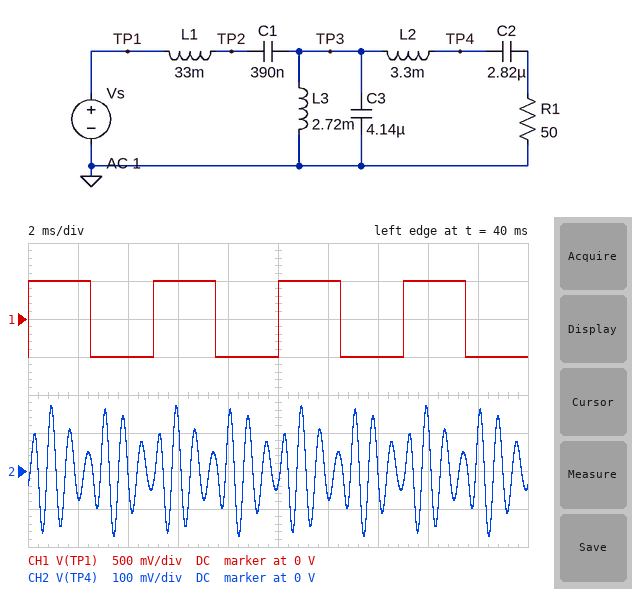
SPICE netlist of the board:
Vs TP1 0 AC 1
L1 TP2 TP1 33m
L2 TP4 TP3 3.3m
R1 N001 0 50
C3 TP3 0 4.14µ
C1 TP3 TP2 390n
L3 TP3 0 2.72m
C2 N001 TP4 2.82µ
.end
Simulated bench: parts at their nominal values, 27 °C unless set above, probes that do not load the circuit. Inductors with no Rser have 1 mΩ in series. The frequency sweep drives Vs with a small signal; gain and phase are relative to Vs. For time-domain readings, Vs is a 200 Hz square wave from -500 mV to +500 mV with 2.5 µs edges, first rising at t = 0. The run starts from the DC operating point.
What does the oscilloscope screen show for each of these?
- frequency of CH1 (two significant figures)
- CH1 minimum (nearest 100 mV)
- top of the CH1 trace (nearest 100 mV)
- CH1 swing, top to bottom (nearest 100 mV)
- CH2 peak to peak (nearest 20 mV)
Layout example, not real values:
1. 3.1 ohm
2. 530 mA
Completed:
1. 200 Hz
2. -500 mV
3. 500 mV
4. 1.0 V
5. 340 mV
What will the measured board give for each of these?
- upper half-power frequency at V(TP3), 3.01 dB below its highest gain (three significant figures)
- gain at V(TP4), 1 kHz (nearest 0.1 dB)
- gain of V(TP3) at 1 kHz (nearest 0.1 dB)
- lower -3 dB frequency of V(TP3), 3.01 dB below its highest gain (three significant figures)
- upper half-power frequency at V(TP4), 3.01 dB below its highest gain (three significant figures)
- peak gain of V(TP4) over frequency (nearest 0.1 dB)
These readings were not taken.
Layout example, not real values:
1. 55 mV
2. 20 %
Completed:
1. 1.56 kHz
2. -11.3 dB
3. -13.1 dB
4. 1.22 kHz
5. 1.55 kHz
6. 2.0 dB
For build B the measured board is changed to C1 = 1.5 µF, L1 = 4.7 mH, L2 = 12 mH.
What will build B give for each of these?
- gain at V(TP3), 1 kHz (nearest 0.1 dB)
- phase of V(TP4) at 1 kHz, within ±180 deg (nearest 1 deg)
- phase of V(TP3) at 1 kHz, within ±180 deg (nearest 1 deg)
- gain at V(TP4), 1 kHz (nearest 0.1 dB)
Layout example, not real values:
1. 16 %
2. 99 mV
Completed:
1. -7.6 dB
2. 77 deg
3. 146 deg
4. -4.6 dB
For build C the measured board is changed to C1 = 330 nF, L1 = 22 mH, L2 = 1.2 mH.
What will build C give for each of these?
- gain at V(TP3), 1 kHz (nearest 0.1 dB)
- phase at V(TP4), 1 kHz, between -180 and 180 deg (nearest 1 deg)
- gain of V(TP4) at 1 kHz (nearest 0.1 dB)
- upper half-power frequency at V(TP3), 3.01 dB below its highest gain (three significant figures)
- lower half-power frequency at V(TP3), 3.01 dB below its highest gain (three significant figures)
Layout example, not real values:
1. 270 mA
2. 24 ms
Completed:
1. -17.6 dB
2. 148 deg
3. -17.0 dB
4. 2.03 kHz
5. 1.90 kHz
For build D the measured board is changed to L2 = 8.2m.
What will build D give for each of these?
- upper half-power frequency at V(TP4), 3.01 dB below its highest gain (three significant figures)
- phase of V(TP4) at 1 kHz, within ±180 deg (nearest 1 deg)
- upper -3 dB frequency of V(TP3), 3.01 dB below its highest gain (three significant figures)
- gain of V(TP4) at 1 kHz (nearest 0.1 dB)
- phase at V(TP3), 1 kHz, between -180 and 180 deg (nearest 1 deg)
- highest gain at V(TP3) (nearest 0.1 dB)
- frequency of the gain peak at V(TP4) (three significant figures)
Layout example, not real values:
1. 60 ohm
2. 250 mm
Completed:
1. 1.38 kHz
2. 99 deg
3. 1.39 kHz
4. -12.7 dB
5. 142 deg
6. 3.5 dB
7. 1.32 kHz
